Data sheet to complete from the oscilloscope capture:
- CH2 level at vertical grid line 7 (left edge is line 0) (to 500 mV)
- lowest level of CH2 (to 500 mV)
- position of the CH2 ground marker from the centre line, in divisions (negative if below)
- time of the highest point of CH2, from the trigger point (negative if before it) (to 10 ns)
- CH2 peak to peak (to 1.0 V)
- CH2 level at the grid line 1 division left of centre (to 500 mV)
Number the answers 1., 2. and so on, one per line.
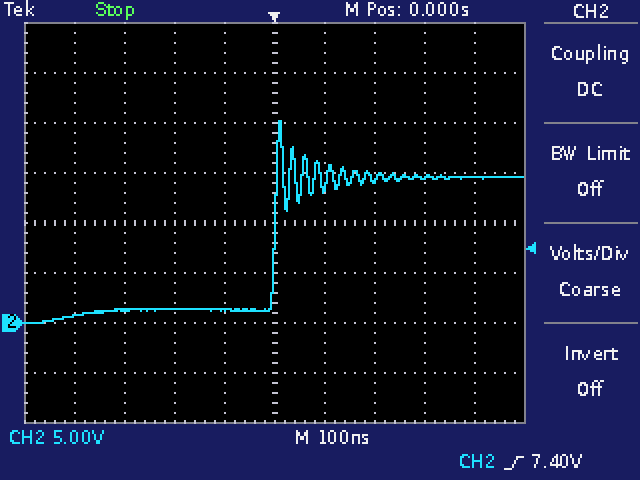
1. 14.5 V
2. 0.0 V
3. -2.0 div
4. +10 ns
5. 20.0 V
6. 1.5 V
